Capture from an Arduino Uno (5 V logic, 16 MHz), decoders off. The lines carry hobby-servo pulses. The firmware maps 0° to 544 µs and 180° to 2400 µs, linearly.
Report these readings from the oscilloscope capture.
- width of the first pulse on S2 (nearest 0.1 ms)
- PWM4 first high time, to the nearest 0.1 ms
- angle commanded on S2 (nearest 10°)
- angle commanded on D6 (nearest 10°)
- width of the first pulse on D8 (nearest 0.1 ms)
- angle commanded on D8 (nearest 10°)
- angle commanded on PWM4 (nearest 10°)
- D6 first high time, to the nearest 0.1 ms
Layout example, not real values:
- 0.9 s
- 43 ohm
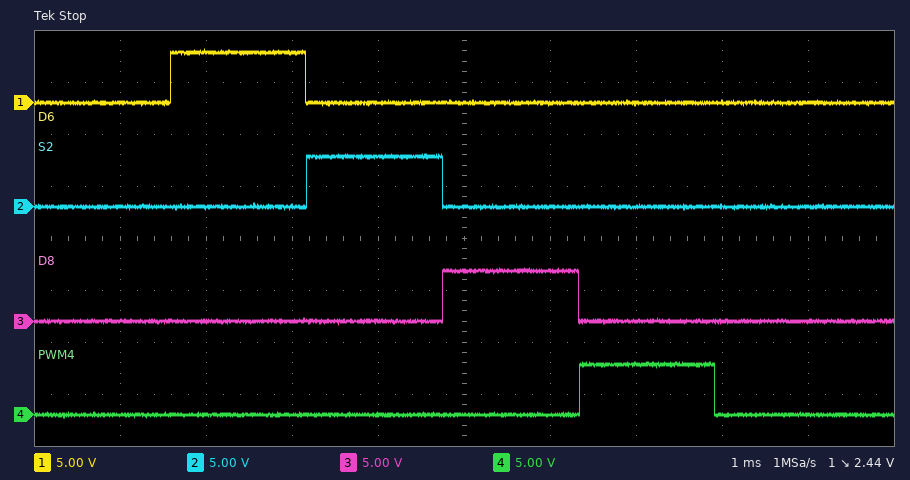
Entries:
- 1.6 ms
- 1.6 ms
- 100°
- 100°
- 1.6 ms
- 100°
- 100°
- 1.6 ms
